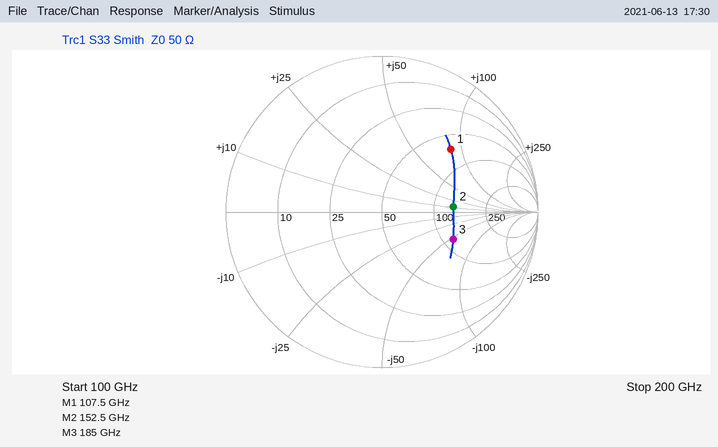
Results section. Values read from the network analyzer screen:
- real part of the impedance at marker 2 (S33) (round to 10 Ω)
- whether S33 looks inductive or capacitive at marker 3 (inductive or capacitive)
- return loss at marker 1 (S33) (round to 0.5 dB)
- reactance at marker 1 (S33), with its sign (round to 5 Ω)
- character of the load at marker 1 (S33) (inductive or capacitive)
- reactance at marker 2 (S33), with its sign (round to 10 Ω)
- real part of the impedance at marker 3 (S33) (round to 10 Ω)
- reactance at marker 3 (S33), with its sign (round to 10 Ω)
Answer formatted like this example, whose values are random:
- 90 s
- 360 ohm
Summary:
- 130 Ω
- capacitive
- 4.5 dB
- +85 Ω
- inductive
- +10 Ω
- 120 Ω
- -50 Ω
